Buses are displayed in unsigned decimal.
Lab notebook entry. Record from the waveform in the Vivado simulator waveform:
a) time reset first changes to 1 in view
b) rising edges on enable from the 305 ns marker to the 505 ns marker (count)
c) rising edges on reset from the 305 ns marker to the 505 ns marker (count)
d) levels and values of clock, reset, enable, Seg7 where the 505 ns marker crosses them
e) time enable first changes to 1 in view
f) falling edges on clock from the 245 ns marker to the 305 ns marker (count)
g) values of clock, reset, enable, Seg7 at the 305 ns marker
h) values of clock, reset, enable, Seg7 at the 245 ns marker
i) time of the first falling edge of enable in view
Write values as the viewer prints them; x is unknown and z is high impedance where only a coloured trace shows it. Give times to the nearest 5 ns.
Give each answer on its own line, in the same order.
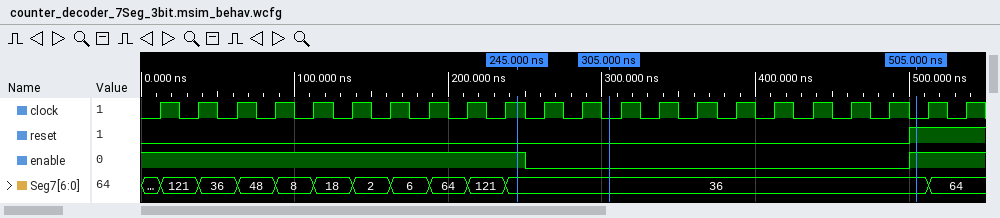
500 ns
1
1
clock=0, reset=1, enable=1, Seg7=36
500 ns
3
clock=0, reset=0, enable=0, Seg7=36
clock=1, reset=0, enable=1, Seg7=36
250 ns
